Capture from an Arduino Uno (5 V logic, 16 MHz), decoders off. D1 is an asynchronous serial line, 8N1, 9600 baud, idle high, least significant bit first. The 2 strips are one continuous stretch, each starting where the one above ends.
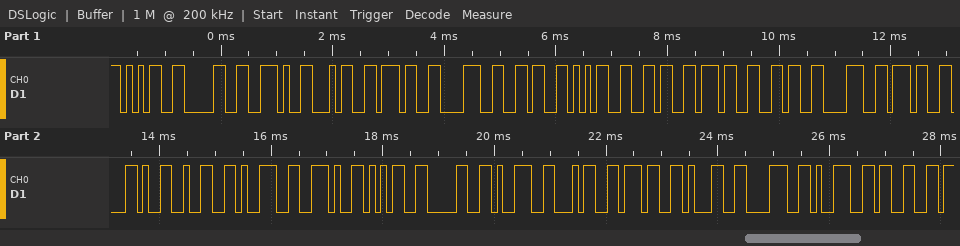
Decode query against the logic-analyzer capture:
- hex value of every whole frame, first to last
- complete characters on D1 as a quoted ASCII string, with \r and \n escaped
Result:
0x35 0x30 0x2E 0x34 0x37 0x38 0x36 0x35 0x36 0x37 0x36 0x38 0x37 0x2C 0x32 0x39 0x2E 0x35 0x30 0x39 0x34 0x37 0x31 0x38 0x39 0x33
"50.4786567687,29.509471893"
